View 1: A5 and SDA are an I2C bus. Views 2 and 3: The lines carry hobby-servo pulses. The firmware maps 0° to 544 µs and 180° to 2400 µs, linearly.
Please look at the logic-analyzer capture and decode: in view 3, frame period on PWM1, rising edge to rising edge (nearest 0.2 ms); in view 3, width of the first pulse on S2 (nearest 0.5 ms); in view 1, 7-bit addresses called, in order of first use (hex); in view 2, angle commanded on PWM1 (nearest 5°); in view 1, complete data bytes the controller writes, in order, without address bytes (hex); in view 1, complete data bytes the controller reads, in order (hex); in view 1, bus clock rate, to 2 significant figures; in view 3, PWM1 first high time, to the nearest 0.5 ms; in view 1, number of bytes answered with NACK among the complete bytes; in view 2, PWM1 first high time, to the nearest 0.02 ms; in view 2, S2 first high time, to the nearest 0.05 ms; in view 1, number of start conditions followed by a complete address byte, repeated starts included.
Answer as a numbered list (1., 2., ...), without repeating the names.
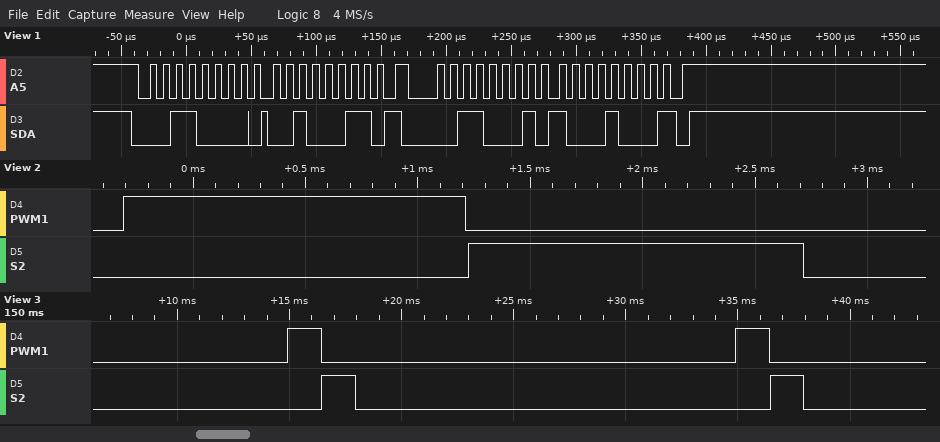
1. 20.0 ms
2. 1.5 ms
3. 0x18
4. 95°
5. 23
6. 88
7. 100 kHz
8. 1.5 ms
9. 1
10. 1.52 ms
11. 1.50 ms
12. 2
